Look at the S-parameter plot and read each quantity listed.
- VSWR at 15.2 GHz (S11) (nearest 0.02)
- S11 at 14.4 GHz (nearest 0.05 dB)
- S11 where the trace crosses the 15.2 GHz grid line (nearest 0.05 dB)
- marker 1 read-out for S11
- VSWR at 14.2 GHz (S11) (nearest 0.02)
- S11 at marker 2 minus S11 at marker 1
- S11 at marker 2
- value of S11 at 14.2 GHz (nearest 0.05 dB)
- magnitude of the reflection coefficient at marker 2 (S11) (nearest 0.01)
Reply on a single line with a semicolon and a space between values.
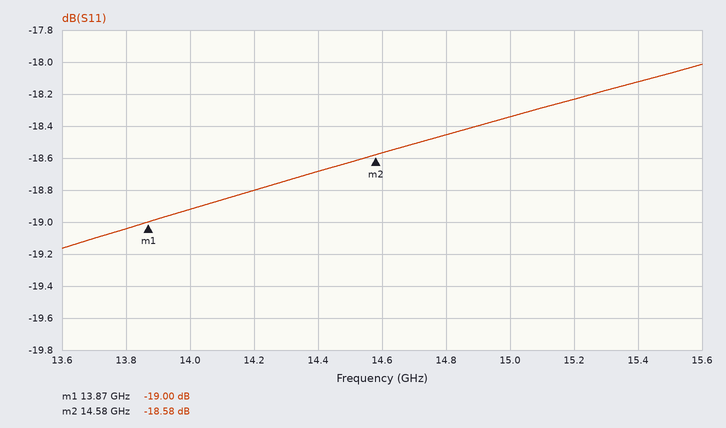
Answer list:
1.28; -18.70 dB; -18.25 dB; -19.00 dB; 1.26; 0.42 dB; -18.58 dB; -18.80 dB; 0.12
